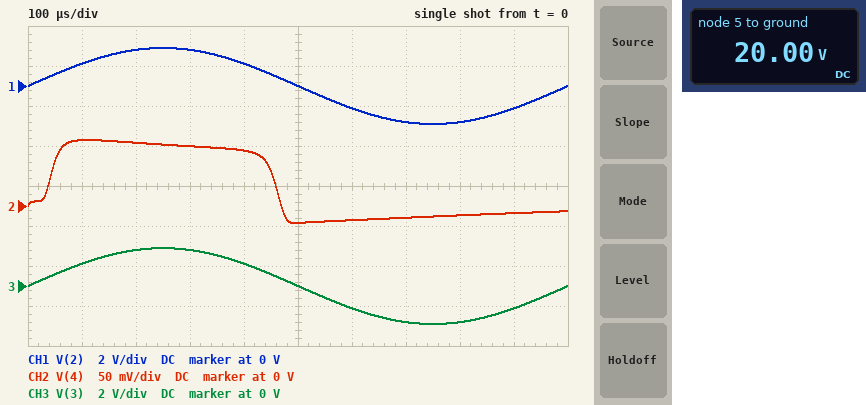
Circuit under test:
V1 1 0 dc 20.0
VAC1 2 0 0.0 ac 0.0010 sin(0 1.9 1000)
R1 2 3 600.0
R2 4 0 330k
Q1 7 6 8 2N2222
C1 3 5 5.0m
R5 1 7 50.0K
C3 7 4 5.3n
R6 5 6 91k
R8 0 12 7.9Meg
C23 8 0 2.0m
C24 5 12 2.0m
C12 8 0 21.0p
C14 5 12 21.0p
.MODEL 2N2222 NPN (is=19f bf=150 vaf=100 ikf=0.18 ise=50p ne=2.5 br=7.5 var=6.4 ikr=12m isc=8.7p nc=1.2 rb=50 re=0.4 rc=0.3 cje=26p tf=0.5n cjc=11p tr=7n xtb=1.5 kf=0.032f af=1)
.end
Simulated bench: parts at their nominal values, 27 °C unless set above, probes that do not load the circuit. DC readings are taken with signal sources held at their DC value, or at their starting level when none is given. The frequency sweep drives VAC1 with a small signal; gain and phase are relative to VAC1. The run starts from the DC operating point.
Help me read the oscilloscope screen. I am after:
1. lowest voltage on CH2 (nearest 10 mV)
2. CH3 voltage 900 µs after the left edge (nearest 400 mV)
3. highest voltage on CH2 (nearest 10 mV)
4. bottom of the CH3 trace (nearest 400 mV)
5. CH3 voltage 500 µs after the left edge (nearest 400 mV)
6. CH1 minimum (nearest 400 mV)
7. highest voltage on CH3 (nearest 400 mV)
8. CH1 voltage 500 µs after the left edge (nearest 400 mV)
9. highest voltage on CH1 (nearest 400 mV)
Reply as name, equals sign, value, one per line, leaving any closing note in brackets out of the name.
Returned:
lowest voltage on CH2 = -20 mV
CH3 voltage 900 µs after the left edge = -1.2 V
highest voltage on CH2 = 80 mV
bottom of the CH3 trace = -2.0 V
CH3 voltage 500 µs after the left edge = 0 V
CH1 minimum = -2.0 V
highest voltage on CH3 = 2.0 V
CH1 voltage 500 µs after the left edge = 0 V
highest voltage on CH1 = 2.0 V
